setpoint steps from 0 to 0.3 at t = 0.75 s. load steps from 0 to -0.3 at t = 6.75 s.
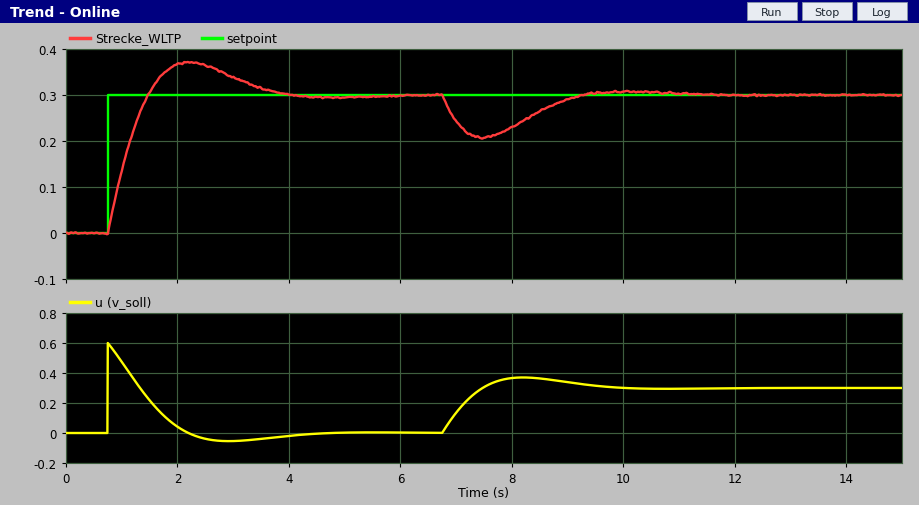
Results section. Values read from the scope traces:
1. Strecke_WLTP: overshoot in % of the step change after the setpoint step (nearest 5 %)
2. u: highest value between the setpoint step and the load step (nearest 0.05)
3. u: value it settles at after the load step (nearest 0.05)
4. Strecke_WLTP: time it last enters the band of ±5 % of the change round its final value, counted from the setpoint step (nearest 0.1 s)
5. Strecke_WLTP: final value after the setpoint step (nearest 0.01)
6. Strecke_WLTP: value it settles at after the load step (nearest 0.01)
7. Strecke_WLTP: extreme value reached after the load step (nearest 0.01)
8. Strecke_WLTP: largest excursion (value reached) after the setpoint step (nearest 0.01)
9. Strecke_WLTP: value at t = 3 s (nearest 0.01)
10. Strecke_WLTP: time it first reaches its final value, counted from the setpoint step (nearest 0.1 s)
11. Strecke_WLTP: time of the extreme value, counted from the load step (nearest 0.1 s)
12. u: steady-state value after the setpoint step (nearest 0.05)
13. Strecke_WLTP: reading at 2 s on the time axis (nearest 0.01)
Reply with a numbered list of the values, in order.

1. 25 %
2. 0.60
3. 0.30
4. 2.8 s
5. 0.30
6. 0.30
7. 0.21
8. 0.37
9. 0.34
10. 0.7 s
11. 0.7 s
12. 0.00
13. 0.37
